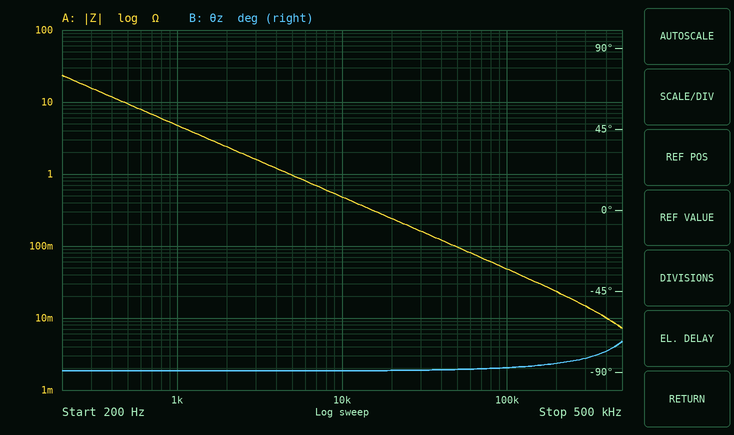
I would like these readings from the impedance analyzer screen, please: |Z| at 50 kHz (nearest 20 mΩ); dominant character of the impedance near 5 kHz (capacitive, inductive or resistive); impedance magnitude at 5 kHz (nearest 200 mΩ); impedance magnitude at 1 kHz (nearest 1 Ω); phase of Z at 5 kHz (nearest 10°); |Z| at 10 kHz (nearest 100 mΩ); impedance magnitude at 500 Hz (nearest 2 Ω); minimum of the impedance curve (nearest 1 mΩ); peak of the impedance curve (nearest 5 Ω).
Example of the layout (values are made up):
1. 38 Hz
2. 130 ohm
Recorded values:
1. 100 mΩ
2. capacitive
3. 1.0 Ω
4. 5 Ω
5. -90°
6. 500 mΩ
7. 10 Ω
8. 7 mΩ
9. 25 Ω
